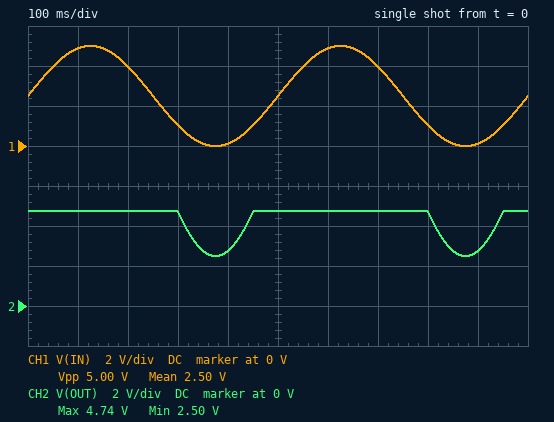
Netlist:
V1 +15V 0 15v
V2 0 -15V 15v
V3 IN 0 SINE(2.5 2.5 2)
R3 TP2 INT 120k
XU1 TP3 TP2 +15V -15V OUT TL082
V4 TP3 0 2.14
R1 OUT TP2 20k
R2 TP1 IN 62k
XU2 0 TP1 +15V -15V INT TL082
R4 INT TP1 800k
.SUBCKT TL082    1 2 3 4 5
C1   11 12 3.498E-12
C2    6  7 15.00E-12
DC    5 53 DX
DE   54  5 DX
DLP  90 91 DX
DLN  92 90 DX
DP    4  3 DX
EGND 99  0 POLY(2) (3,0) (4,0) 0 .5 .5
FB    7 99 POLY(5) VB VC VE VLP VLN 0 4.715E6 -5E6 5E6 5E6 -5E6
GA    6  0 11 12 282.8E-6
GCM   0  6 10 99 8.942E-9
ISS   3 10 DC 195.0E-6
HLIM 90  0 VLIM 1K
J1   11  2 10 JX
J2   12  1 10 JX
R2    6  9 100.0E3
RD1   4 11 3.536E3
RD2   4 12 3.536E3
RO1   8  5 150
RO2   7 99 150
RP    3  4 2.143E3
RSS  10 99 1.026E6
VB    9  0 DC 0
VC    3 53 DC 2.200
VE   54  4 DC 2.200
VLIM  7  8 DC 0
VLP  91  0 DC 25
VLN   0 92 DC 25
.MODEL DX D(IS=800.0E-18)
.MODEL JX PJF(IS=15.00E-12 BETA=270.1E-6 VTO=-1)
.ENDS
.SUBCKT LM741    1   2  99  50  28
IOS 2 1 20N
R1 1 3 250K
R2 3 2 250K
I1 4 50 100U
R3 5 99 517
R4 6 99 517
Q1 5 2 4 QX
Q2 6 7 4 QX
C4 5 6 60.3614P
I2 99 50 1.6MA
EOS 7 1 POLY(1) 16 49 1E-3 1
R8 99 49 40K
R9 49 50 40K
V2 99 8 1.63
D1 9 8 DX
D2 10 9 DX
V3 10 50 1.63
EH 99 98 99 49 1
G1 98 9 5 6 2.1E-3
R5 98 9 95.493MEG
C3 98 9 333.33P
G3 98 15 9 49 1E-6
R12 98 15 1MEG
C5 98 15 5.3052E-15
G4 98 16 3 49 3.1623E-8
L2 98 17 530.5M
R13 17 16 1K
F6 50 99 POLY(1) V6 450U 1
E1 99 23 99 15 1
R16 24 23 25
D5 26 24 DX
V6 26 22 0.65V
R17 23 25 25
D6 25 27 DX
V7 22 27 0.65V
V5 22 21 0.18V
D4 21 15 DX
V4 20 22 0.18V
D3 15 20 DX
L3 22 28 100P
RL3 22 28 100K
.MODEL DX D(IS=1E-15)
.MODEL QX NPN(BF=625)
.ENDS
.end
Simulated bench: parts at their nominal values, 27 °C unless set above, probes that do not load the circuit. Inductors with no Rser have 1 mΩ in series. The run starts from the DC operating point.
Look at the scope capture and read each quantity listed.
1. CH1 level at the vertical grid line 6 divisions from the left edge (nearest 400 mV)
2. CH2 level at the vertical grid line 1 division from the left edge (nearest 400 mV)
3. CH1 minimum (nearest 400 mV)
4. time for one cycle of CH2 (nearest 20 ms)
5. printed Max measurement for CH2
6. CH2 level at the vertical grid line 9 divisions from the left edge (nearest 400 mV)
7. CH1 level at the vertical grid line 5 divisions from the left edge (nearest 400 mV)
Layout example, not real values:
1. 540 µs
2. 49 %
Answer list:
1. 4.8 V
2. 4.8 V
3. 0 V
4. 500 ms
5. 4.74 V
6. 2.8 V
7. 2.4 V
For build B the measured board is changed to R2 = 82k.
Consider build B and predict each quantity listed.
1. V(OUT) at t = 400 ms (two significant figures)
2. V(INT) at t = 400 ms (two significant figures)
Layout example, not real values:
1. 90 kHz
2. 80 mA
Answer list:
1. 2.7 V
2. -1.2 V
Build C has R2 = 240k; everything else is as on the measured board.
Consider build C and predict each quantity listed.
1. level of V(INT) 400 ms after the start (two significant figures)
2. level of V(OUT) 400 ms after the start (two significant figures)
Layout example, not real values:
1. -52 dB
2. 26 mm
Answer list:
1. -410 mV
2. 2.6 V
